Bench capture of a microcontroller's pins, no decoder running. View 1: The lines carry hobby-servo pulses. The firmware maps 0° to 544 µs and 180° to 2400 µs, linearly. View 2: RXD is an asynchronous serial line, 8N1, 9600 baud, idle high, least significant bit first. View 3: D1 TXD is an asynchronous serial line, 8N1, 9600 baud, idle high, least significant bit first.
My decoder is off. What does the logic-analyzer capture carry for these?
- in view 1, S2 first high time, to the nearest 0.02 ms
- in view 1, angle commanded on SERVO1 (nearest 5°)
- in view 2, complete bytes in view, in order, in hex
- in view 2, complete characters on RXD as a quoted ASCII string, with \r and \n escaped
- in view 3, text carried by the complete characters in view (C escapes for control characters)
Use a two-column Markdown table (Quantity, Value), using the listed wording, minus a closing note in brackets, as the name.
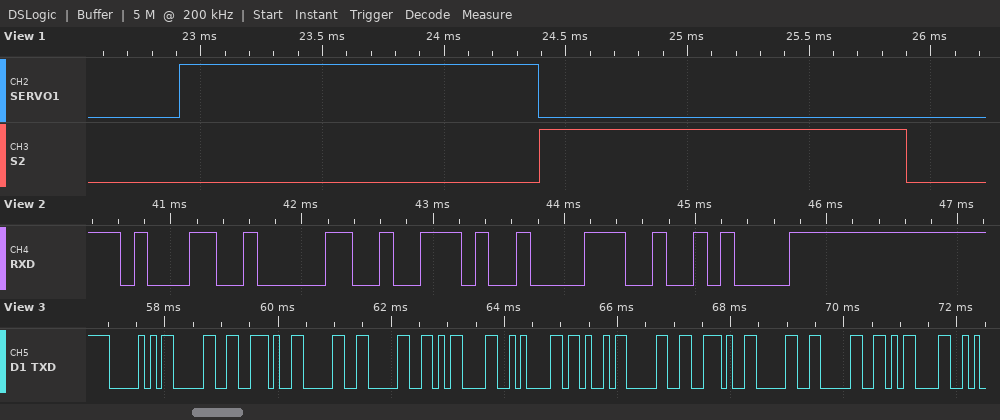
| Quantity | Value |
|---|---|
| in view 1, S2 first high time, to the nearest 0.02 ms | 1.50 ms |
| in view 1, angle commanded on SERVO1 | 90° |
| in view 2, complete bytes in view, in order, in hex | 31 30 2E 38 0A |
| in view 2, complete characters on RXD as a quoted ASCII string, with \r and \n escaped | "10.8\n" |
| in view 3, text carried by the complete characters in view | "P0.00\r\nK0.00\r" |
